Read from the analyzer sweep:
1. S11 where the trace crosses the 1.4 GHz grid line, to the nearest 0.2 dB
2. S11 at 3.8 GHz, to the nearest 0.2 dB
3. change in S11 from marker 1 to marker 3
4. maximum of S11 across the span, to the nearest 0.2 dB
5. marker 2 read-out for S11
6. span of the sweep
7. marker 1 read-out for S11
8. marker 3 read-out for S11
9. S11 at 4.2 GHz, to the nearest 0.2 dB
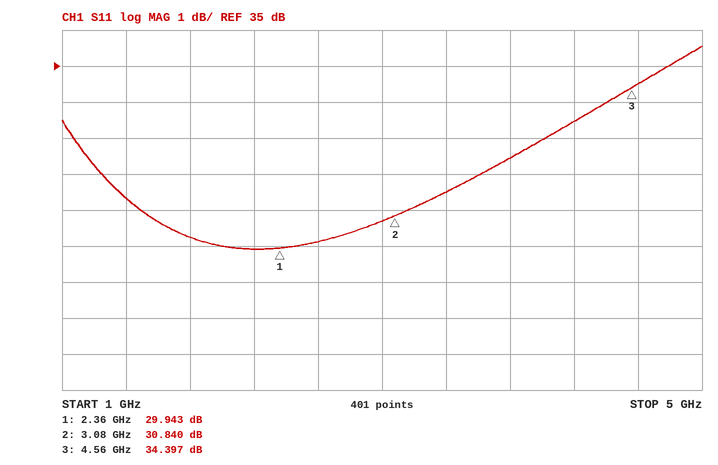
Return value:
31.4 dB
32.4 dB
4.454 dB
35.6 dB
30.840 dB
4 GHz
29.943 dB
34.397 dB
33.4 dB
